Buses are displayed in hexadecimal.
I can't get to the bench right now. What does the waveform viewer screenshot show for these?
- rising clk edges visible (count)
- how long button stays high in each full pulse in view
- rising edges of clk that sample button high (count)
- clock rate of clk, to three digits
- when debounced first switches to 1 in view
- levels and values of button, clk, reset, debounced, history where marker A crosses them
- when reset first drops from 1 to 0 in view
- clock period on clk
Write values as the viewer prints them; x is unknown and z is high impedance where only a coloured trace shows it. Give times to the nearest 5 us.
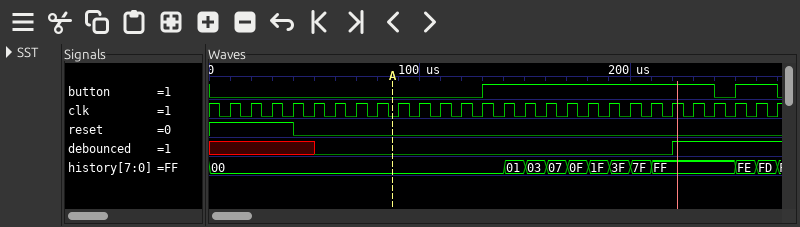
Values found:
27
110 us, 20 us
13
100 kHz
220 us
button=0, clk=0, reset=0, debounced=0, history=00
40 us
10 us
